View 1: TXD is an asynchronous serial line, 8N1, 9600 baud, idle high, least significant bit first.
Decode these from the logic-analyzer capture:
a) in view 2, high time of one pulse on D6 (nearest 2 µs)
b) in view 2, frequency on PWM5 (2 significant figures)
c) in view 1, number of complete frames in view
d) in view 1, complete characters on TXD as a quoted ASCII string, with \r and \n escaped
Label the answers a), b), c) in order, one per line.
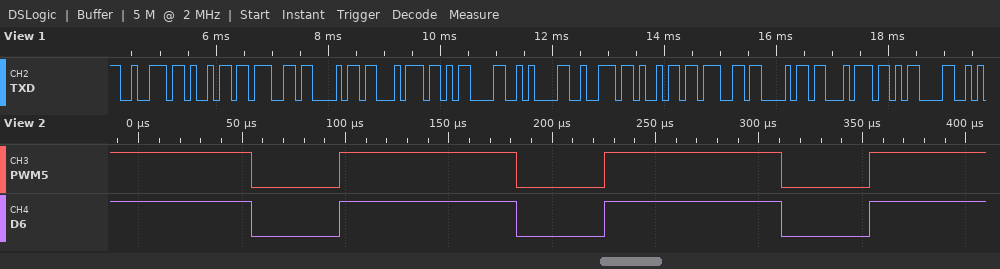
a) 86 µs
b) 7.8 kHz
c) 13
d) "right\r\nright\r"
